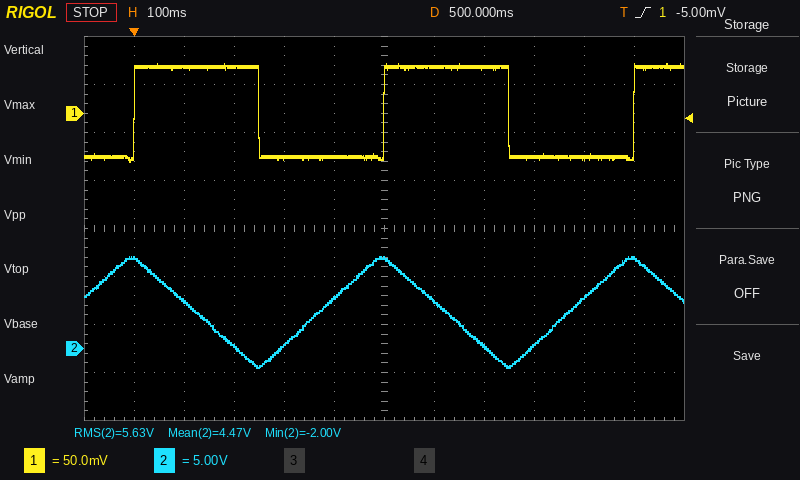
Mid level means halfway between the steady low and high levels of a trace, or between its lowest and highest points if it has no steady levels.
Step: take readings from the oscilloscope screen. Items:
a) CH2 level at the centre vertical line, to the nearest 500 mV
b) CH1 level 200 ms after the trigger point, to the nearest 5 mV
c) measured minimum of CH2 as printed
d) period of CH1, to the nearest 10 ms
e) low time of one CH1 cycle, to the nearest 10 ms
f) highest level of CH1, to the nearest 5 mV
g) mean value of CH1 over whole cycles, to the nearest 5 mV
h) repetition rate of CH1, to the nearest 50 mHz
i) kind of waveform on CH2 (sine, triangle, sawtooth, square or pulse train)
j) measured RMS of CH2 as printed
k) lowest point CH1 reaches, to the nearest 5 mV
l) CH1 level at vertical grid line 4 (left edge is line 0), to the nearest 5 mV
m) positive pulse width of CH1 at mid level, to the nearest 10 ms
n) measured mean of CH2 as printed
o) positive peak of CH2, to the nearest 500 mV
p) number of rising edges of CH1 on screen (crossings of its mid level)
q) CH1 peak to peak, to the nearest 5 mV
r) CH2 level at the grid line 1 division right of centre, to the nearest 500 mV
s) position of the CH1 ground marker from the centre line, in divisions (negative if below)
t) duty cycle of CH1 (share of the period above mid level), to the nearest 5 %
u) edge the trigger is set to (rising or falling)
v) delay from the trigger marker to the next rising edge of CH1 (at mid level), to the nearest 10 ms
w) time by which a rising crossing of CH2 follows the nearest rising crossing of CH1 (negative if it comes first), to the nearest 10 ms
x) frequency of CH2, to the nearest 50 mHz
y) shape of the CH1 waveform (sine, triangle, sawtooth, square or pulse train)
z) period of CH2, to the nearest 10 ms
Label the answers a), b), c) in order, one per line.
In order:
a) 9.5 V
b) 50 mV
c) -2.00 V
d) 500 ms
e) 250 ms
f) 50 mV
g) 0 mV
h) 2.00 Hz
i) triangle
j) 5.63 V
k) -50 mV
l) -45 mV
m) 250 ms
n) 4.47 V
o) 9.5 V
p) 3
q) 100 mV
r) 5.0 V
s) +2.4 div
t) 50 %
u) rising
v) 500 ms
w) -130 ms
x) 2.00 Hz
y) square
z) 500 ms
